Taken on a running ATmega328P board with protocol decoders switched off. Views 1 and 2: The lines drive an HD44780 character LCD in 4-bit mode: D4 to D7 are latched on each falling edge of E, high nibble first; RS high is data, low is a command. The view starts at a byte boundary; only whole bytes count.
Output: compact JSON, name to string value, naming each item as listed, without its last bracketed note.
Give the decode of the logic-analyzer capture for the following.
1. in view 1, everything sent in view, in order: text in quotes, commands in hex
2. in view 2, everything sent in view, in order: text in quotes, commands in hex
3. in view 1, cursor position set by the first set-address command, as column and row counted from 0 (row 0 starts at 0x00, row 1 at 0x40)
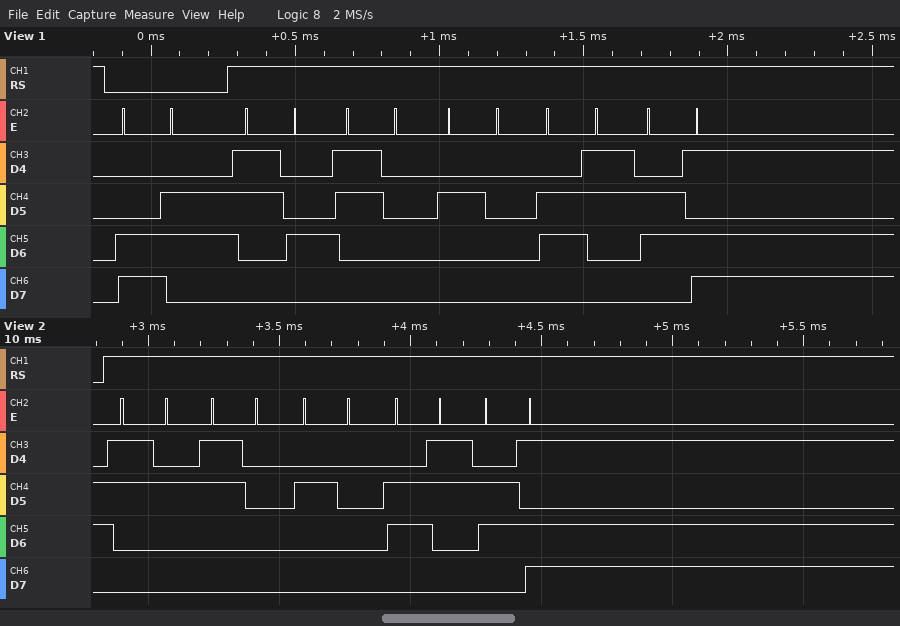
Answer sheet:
{"in view 1, everything sent in view, in order: text in quotes, commands in hex": "0xC6 \"40 cm\"", "in view 2, everything sent in view, in order: text in quotes, commands in hex": "\"20 cm\"", "in view 1, cursor position set by the first set-address command, as column and row counted from 0": "column 6, row 1"}
